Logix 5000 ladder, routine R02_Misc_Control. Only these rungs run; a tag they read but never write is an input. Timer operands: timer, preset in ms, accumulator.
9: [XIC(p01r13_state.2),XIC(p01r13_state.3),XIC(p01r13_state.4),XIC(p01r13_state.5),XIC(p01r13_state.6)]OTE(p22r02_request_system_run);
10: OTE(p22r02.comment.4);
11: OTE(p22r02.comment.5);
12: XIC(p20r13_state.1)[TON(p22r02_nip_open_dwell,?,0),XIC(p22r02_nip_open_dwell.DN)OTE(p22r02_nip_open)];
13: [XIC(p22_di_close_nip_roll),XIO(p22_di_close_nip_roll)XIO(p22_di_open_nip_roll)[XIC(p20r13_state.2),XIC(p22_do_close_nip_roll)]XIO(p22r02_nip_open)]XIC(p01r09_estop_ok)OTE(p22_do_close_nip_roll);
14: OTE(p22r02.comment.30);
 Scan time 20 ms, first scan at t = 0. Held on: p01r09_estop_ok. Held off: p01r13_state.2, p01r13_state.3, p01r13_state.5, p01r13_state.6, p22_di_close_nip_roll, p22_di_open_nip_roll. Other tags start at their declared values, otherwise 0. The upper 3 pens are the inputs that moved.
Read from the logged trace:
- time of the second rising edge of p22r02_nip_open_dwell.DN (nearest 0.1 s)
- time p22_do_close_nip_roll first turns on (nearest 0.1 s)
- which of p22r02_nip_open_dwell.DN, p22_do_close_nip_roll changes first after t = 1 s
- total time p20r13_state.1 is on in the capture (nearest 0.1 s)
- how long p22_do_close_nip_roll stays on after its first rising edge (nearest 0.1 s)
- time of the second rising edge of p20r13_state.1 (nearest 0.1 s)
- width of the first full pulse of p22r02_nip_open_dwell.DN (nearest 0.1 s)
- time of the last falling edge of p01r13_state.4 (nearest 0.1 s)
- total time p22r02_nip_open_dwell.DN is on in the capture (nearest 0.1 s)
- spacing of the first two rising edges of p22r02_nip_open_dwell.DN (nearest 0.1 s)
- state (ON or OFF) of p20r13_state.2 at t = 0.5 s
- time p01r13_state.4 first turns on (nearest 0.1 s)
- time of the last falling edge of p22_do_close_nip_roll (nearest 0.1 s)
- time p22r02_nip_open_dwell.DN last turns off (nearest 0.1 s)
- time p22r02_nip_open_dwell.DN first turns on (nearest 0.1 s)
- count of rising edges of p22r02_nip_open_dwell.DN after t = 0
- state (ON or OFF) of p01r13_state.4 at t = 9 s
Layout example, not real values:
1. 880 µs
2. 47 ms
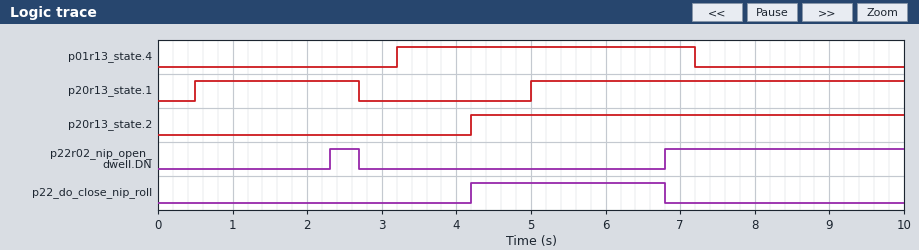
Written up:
1. 6.8 s
2. 4.2 s
3. p22r02_nip_open_dwell.DN
4. 7.2 s
5. 2.6 s
6. 5.0 s
7. 0.4 s
8. 7.2 s
9. 3.6 s
10. 4.5 s
11. OFF
12. 3.2 s
13. 6.8 s
14. 2.7 s
15. 2.3 s
16. 2
17. OFF
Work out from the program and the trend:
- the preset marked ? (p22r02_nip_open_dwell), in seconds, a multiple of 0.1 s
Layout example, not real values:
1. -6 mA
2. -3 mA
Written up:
1. 1.8 s
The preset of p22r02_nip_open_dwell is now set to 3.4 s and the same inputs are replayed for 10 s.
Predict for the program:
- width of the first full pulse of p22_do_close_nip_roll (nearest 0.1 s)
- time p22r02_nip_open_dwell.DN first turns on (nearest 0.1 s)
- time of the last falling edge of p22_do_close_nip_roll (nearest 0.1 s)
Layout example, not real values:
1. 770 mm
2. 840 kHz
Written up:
1. 4.2 s
2. 8.4 s
3. 8.4 s
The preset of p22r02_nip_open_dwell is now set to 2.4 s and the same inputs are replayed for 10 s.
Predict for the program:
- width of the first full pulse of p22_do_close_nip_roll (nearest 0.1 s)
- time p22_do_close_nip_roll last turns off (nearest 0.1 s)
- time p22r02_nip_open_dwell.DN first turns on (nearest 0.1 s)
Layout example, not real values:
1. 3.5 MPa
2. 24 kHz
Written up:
1. 3.2 s
2. 7.4 s
3. 7.4 s
